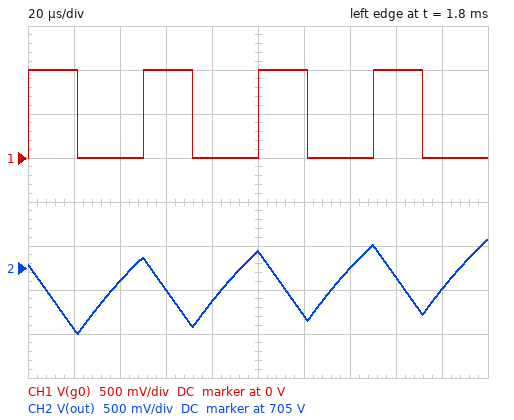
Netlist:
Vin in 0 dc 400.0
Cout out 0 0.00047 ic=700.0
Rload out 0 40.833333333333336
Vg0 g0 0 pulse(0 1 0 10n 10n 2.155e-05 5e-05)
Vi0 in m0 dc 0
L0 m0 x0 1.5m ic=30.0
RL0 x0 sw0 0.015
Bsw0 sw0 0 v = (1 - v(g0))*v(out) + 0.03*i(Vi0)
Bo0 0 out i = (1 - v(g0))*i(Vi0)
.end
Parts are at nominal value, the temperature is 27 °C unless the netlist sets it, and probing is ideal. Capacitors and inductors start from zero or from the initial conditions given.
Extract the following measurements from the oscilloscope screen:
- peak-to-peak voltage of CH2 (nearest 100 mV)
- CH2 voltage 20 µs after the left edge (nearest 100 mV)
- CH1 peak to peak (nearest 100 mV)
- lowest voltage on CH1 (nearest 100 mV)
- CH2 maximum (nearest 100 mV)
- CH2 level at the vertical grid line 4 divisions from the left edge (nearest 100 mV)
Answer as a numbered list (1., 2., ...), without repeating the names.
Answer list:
1. 1.1 V
2. 704.3 V
3. 1.0 V
4. 0 V
5. 705.3 V
6. 704.6 V
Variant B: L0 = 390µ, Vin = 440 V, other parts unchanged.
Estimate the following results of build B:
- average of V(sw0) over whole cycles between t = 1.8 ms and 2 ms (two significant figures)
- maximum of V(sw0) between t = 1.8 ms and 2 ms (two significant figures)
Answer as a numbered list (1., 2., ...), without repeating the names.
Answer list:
1. 470 V
2. 830 V
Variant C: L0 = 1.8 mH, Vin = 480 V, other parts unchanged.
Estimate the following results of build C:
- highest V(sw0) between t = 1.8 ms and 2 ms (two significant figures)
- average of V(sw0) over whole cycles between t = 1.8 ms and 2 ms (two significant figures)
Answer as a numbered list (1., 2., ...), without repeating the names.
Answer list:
1. 800 V
2. 450 V
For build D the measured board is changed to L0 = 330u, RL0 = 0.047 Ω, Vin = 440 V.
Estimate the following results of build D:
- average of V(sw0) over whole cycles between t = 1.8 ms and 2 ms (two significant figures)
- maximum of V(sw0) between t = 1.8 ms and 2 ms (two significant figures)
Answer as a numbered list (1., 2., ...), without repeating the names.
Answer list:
1. 470 V
2. 820 V
